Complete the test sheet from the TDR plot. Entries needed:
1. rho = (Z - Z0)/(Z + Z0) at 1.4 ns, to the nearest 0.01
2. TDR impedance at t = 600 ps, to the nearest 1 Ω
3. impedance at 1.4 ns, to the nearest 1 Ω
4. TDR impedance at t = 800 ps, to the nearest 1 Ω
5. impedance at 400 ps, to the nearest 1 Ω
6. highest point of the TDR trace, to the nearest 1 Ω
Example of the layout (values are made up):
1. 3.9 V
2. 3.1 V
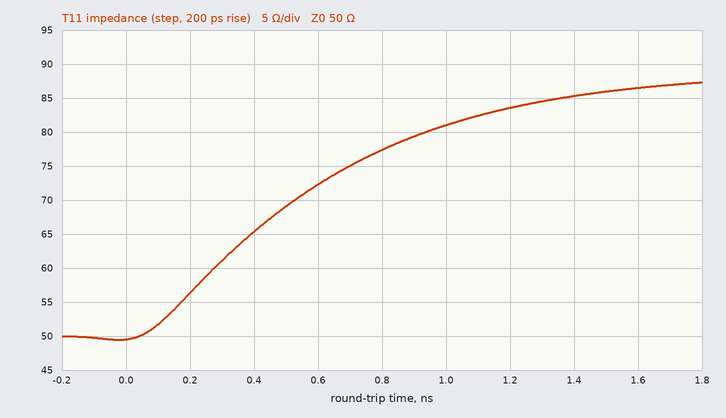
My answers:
1. +0.26
2. 72 Ω
3. 85 Ω
4. 77 Ω
5. 65 Ω
6. 87 Ω
